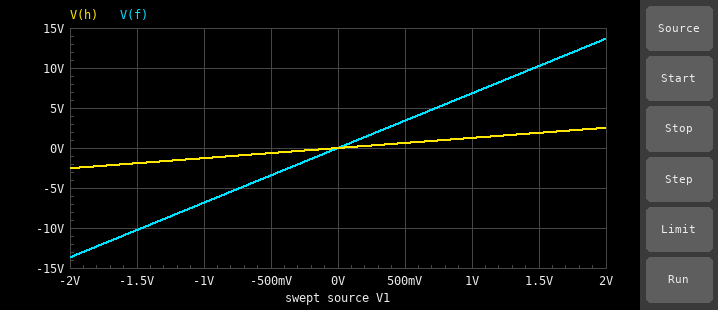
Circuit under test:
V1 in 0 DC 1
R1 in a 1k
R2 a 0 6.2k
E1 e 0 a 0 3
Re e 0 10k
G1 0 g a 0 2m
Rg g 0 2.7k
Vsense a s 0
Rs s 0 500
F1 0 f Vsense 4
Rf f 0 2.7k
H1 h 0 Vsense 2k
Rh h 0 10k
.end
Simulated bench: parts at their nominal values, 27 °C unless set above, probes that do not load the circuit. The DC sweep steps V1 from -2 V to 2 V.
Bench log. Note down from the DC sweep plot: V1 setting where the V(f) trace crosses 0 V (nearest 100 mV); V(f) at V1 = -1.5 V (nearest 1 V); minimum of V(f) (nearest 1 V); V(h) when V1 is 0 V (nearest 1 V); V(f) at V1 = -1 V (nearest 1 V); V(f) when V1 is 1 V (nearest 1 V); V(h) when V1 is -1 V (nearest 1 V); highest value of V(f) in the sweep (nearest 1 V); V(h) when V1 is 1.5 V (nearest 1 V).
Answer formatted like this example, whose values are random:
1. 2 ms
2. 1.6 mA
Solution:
1. 0 V
2. -10 V
3. -14 V
4. 0 V
5. -7 V
6. 7 V
7. -1 V
8. 14 V
9. 2 V
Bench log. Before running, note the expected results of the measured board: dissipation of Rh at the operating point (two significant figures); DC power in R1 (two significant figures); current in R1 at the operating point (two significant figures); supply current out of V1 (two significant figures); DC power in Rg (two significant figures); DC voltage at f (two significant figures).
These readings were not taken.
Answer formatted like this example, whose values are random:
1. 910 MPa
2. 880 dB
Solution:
1. 160 µW
2. 470 µW
3. 680 µA
4. 680 µA
5. 1.1 mW
6. 6.8 V
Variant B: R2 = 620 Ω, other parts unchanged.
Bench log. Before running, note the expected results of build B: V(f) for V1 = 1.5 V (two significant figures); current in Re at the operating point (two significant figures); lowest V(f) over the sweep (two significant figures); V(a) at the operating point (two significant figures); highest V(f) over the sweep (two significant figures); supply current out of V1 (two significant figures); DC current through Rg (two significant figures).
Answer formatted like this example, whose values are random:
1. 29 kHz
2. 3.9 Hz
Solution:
1. 7.0 V
2. 65 µA
3. -9.4 V
4. 220 mV
5. 9.4 V
6. 780 µA
7. 430 µA
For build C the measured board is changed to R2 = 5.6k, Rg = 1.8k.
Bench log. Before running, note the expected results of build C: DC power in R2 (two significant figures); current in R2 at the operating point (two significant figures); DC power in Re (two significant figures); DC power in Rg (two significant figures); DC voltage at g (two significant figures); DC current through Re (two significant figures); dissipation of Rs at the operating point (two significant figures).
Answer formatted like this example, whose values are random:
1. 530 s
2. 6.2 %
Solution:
1. 18 µW
2. 56 µA
3. 89 µW
4. 710 µW
5. 1.1 V
6. 94 µA
7. 200 µW
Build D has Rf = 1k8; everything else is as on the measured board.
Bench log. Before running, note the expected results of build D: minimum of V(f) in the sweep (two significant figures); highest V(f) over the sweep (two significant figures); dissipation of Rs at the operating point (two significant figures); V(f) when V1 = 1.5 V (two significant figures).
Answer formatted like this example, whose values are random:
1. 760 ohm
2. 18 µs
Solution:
1. -9.1 V
2. 9.1 V
3. 200 µW
4. 6.8 V
